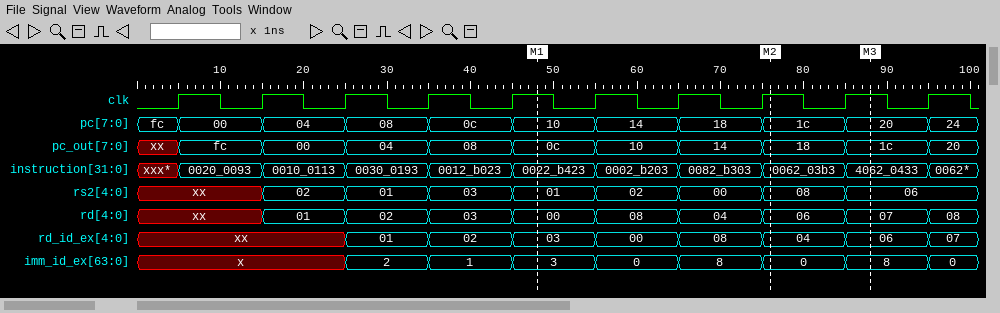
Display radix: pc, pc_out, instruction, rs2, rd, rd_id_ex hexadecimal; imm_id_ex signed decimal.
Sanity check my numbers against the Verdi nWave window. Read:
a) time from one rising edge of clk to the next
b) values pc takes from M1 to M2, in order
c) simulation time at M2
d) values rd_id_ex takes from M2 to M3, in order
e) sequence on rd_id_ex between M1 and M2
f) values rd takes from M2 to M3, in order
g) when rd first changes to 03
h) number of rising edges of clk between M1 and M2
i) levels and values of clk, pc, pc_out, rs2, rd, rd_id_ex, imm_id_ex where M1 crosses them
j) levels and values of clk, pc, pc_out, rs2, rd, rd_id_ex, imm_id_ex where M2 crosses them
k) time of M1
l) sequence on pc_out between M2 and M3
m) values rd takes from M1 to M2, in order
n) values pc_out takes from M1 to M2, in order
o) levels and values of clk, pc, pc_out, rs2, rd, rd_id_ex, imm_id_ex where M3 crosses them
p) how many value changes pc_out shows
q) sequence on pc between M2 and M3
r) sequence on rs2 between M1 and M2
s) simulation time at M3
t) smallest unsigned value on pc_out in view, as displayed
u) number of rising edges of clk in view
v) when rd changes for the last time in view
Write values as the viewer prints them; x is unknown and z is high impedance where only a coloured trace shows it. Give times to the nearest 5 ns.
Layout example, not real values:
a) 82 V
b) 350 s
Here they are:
a) 10 ns
b) 10, 14, 18, 1c
c) 75 ns
d) 04, 06
e) 03, 00, 08, 04
f) 06, 07
g) 35 ns
h) 3
i) clk=1, pc=10, pc_out=0c, rs2=01, rd=00, rd_id_ex=03, imm_id_ex=3
j) clk=1, pc=1c, pc_out=18, rs2=08, rd=06, rd_id_ex=04, imm_id_ex=0
k) 50 ns
l) 18, 1c
m) 00, 08, 04, 06
n) 0c, 10, 14, 18
o) clk=1, pc=20, pc_out=1c, rs2=06, rd=07, rd_id_ex=06, imm_id_ex=8
p) 10
q) 1c, 20
r) 01, 02, 00, 08
s) 90 ns
t) 00
u) 10
v) 95 ns
